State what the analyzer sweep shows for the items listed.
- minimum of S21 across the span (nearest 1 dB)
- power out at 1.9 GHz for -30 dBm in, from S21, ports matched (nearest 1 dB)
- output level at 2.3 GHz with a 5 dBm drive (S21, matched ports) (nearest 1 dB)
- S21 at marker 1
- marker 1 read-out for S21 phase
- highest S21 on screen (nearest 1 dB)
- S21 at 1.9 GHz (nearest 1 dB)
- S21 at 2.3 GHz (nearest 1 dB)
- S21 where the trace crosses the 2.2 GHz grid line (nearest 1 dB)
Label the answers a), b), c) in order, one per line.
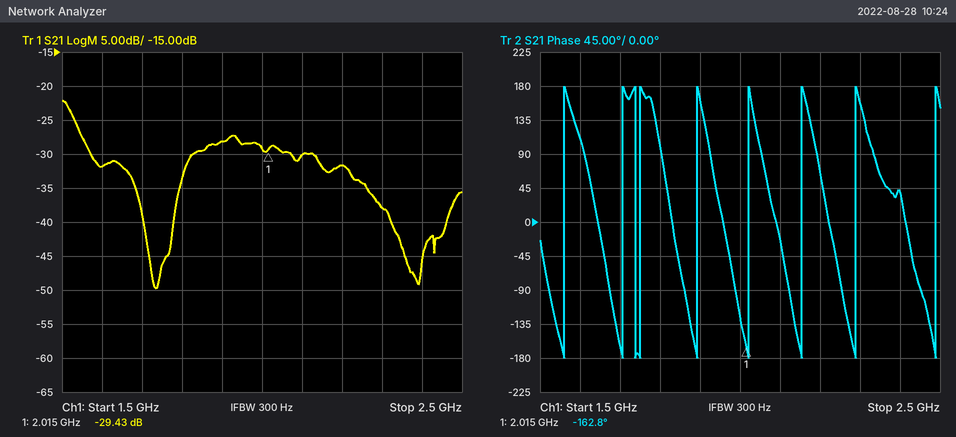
a) -50 dB
b) -58 dBm
c) -33 dBm
d) -29.43 dB
e) -162.8°
f) -22 dB
g) -28 dB
h) -38 dB
i) -32 dB
